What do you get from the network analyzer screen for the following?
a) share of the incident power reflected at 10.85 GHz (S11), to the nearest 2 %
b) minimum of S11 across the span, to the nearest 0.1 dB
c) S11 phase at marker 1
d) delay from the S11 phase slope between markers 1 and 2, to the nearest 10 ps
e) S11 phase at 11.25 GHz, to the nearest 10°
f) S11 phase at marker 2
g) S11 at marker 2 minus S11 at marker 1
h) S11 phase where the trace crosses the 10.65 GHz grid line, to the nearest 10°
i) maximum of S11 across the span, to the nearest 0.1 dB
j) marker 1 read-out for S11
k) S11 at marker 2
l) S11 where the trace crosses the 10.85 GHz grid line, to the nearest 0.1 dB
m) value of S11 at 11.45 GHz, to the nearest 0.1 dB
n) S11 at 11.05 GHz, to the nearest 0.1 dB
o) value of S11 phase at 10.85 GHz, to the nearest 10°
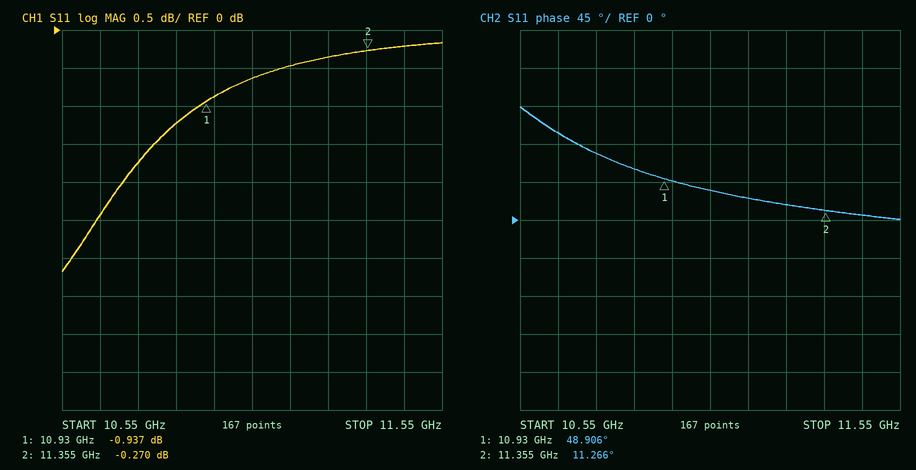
76 %
-3.2 dB
48.906°
250 ps
20°
11.266°
0.667 dB
100°
-0.2 dB
-0.937 dB
-0.270 dB
-1.2 dB
-0.2 dB
-0.6 dB
60°
